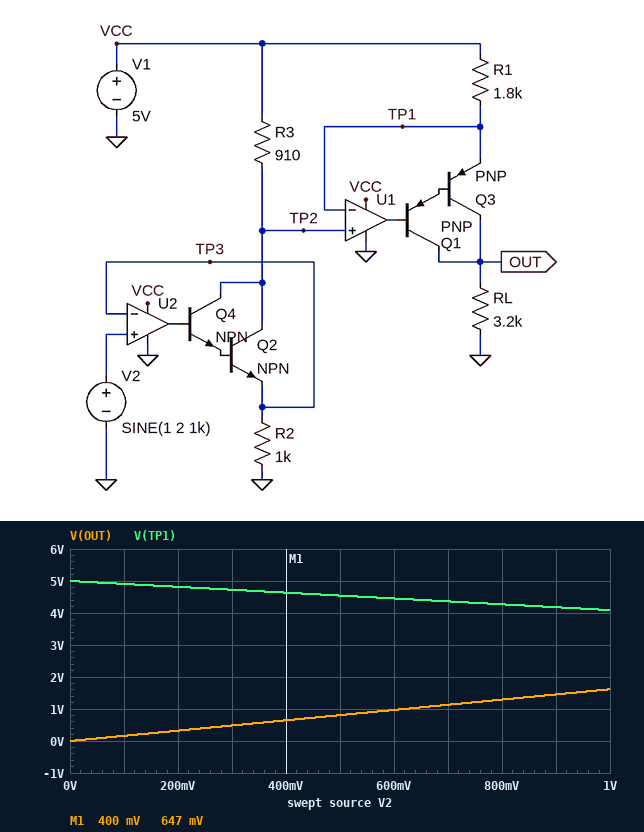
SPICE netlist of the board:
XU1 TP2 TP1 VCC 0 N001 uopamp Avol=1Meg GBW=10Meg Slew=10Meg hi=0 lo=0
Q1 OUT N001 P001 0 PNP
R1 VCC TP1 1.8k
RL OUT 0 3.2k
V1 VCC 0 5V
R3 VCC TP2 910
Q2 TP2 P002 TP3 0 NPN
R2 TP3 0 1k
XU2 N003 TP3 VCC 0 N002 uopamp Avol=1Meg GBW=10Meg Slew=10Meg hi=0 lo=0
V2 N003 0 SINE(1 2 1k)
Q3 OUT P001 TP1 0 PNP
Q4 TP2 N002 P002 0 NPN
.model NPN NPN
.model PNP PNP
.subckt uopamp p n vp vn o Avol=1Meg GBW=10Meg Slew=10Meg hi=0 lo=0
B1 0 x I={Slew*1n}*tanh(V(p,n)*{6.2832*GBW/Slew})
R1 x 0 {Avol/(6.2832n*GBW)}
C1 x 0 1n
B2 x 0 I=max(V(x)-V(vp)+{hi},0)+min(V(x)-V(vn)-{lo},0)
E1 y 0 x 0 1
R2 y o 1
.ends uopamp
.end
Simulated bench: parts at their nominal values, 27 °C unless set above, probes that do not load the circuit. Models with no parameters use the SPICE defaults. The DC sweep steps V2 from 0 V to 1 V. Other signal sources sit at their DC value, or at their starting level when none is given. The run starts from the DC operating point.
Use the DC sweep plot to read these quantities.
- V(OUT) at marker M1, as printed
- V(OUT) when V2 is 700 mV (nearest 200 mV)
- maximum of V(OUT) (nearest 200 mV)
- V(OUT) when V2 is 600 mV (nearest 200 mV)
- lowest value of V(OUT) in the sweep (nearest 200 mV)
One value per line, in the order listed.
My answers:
647 mV
1.2 V
1.6 V
1.0 V
0 V
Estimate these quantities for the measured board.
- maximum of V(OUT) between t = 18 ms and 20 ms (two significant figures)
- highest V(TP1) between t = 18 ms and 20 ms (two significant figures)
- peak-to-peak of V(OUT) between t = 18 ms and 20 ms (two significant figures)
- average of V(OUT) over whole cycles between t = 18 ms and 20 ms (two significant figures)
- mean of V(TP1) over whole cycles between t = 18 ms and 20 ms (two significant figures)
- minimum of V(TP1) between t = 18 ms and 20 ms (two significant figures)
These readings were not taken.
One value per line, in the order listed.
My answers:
2.7 V
5.0 V
2.7 V
1.3 V
4.2 V
3.0 V
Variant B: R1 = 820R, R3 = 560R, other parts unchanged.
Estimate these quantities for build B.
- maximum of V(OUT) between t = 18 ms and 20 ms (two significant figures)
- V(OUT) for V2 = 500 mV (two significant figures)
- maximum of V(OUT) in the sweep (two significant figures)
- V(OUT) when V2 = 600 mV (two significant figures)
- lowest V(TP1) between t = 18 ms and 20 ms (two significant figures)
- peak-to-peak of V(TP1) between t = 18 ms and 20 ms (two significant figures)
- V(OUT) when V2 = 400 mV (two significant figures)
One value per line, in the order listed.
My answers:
3.3 V
1.1 V
2.2 V
1.3 V
3.5 V
1.5 V
870 mV
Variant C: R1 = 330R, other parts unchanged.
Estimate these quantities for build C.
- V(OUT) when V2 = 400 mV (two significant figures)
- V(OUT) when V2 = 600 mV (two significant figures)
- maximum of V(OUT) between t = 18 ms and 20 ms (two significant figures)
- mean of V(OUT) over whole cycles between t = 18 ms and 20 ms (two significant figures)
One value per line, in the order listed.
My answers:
3.5 V
3.7 V
3.8 V
1.8 V
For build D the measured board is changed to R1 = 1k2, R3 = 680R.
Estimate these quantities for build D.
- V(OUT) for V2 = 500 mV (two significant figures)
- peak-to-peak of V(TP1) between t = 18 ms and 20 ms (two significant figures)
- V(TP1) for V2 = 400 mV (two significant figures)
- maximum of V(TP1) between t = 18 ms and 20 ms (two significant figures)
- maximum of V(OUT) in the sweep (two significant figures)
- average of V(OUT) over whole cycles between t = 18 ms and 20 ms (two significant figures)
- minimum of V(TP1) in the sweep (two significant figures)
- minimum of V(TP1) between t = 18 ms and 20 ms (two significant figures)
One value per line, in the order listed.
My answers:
910 mV
1.7 V
4.7 V
5.0 V
1.8 V
1.5 V
4.3 V
3.3 V
